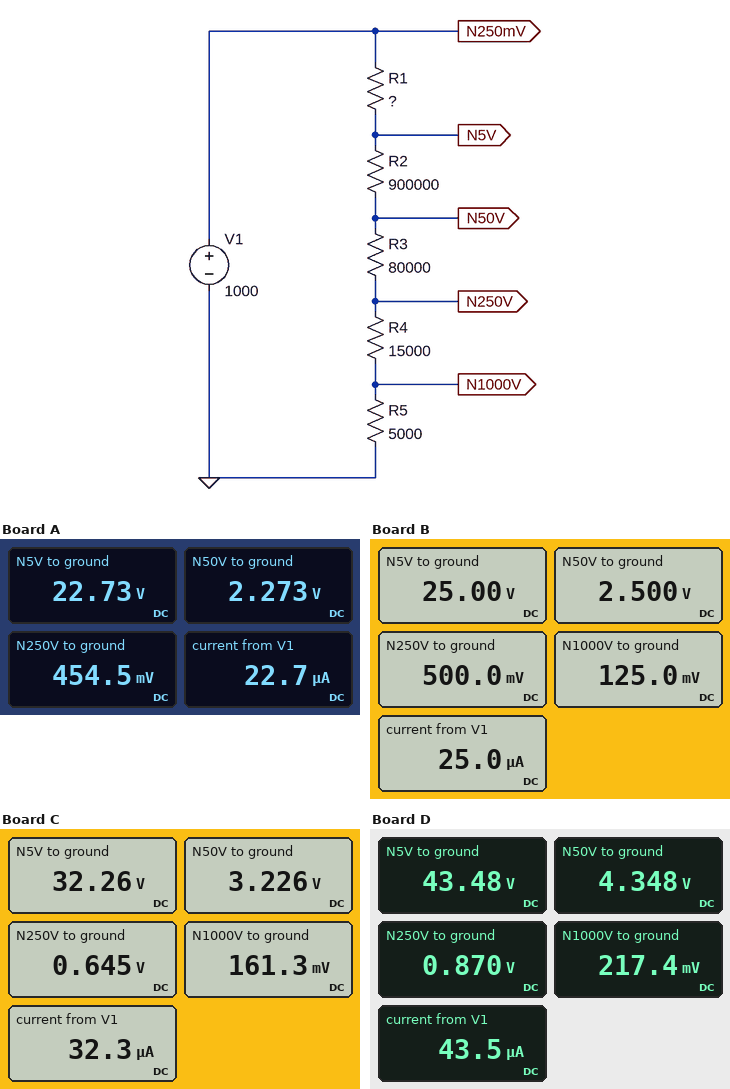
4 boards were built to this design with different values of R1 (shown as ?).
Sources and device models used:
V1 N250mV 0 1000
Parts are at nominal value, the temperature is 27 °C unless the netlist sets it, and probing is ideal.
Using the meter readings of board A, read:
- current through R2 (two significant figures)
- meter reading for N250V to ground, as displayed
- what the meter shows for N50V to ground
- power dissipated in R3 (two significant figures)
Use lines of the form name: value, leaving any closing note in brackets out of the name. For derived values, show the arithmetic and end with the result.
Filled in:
current through R2: (22.73 V - 2.273 V) / 900 kΩ = 23 µA
meter reading for N250V to ground, as displayed: 454.5 mV
what the meter shows for N50V to ground: 2.273 V
power dissipated in R3: (2.273 V - 454.5 mV)^2 / 80 kΩ = 41 µW
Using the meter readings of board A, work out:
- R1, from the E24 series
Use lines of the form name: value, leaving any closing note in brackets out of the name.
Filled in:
R1, from the E24 series: 43 MΩ
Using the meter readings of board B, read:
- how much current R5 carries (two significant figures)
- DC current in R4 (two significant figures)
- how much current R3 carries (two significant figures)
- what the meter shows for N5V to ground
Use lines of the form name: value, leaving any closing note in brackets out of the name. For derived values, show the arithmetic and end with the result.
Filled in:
how much current R5 carries: (125 mV) / 5 kΩ = 25 µA
DC current in R4: (500 mV - 125 mV) / 15 kΩ = 25 µA
how much current R3 carries: (2.5 V - 500 mV) / 80 kΩ = 25 µA
what the meter shows for N5V to ground: 25.00 V
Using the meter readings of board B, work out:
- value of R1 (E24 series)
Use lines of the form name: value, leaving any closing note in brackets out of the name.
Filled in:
value of R1: 39 MΩ
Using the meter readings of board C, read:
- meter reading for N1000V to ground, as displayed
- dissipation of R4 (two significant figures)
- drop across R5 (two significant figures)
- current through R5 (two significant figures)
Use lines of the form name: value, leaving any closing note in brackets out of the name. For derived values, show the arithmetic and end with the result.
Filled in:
meter reading for N1000V to ground, as displayed: 161.3 mV
dissipation of R4: (645 mV - 161.3 mV)^2 / 15 kΩ = 16 µW
drop across R5: 161.3 mV = 160 mV
current through R5: (161.3 mV) / 5 kΩ = 32 µA
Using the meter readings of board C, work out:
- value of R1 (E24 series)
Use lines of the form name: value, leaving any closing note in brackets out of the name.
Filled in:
value of R1: 30 MΩ
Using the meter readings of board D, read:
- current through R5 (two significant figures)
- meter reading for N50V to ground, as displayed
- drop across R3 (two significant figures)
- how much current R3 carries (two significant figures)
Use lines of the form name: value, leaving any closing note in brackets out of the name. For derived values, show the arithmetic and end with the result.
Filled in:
current through R5: (217.4 mV) / 5 kΩ = 43 µA
meter reading for N50V to ground, as displayed: 4.348 V
drop across R3: 4.348 V - 870 mV = 3.5 V
how much current R3 carries: (4.348 V - 870 mV) / 80 kΩ = 43 µA
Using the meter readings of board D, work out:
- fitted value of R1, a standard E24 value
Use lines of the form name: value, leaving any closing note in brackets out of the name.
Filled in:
fitted value of R1, a standard E24 value: 22 MΩ
